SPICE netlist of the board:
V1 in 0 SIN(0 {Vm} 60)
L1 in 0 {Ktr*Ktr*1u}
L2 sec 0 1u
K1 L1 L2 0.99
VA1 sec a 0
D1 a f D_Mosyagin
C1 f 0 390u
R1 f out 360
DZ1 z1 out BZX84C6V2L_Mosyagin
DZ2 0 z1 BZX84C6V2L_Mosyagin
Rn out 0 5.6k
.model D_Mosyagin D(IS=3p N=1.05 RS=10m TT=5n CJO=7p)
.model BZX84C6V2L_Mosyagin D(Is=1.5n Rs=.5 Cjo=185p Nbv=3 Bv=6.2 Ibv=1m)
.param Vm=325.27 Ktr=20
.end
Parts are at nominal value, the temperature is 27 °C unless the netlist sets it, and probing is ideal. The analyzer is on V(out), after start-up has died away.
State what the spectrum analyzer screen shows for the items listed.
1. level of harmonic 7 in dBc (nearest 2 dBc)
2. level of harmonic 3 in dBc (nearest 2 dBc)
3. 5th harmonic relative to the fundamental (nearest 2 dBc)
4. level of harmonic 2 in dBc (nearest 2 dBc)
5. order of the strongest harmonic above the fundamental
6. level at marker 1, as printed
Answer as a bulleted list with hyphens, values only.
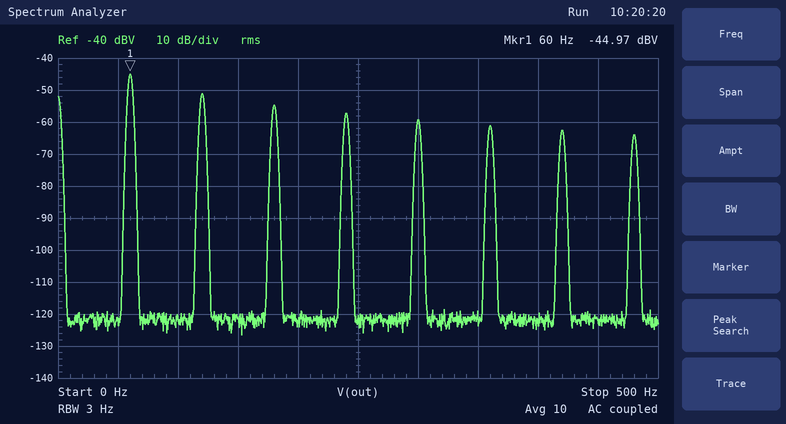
- -18 dBc
- -10 dBc
- -14 dBc
- -6 dBc
- 2
- -44.97 dBV
